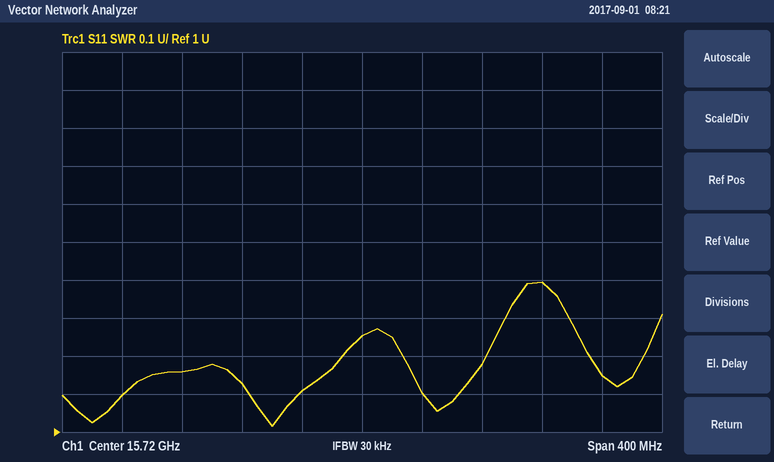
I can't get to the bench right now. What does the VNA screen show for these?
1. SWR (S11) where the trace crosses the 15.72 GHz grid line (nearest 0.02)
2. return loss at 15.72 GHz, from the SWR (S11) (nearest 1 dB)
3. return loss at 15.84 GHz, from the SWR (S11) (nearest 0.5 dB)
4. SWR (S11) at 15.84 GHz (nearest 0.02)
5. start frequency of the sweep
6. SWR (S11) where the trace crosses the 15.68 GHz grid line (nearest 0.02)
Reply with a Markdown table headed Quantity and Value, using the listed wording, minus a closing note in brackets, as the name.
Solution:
| Quantity | Value |
|---|---|
| SWR (S11) where the trace crosses the 15.72 GHz grid line | 1.26 |
| return loss at 15.72 GHz, from the SWR (S11) | 19 dB |
| return loss at 15.84 GHz, from the SWR (S11) | 15.5 dB |
| SWR (S11) at 15.84 GHz | 1.40 |
| start frequency of the sweep | 15.52 GHz |
| SWR (S11) where the trace crosses the 15.68 GHz grid line | 1.10 |
